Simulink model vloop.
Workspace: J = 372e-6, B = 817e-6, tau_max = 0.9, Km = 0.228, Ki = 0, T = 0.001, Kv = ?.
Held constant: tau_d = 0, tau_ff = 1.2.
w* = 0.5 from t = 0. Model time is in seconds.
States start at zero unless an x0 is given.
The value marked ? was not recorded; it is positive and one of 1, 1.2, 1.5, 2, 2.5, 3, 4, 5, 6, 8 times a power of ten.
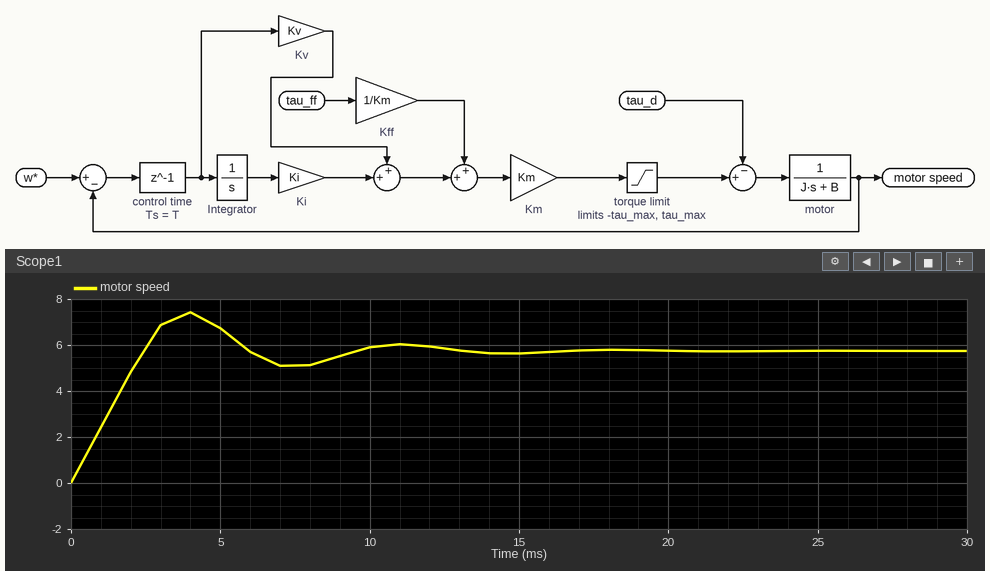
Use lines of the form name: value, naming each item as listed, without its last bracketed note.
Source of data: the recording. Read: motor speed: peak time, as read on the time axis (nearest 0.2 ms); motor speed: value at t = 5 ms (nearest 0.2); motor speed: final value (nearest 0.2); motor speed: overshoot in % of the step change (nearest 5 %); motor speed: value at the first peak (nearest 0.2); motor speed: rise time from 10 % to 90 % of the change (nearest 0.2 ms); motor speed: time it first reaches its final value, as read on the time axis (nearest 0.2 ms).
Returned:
motor speed: peak time, as read on the time axis: 4.0 ms
motor speed: value at t = 5 ms: 6.8
motor speed: final value: 5.8
motor speed: overshoot in % of the step change: 30 %
motor speed: value at the first peak: 7.4
motor speed: rise time from 10 % to 90 % of the change: 2.0 ms
motor speed: time it first reaches its final value, as read on the time axis: 2.4 ms
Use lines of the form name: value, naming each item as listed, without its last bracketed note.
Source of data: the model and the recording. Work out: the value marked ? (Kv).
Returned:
the value marked ?: 1
